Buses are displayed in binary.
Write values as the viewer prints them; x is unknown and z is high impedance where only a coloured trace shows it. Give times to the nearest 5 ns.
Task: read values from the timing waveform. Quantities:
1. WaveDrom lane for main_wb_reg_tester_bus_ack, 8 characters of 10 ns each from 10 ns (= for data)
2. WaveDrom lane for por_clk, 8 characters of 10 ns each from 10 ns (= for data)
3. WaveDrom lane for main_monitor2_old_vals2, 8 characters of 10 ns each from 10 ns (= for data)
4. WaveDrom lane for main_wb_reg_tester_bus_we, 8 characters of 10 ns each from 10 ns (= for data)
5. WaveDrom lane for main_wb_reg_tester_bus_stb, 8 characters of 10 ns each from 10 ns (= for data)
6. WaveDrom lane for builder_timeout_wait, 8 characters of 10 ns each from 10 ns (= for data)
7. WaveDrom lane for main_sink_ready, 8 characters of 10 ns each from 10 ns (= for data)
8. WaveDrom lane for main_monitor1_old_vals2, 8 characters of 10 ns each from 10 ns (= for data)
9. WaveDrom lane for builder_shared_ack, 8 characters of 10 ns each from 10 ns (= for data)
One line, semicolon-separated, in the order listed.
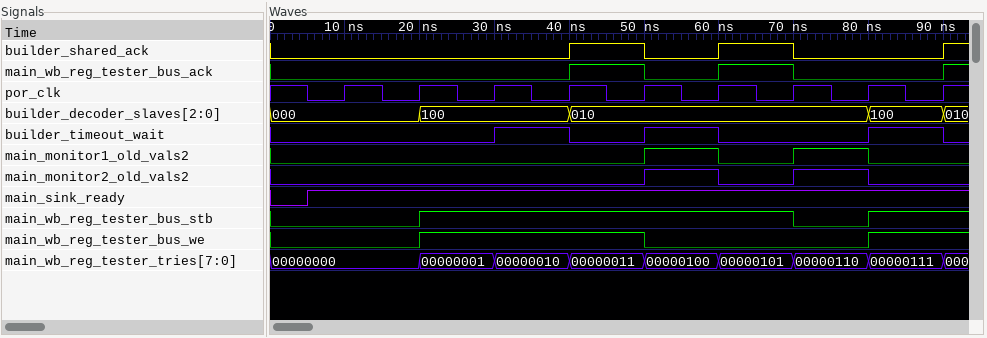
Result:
{name: 'main_wb_reg_tester_bus_ack', wave: '0..1010.'}; {name: 'por_clk', wave: 'p.......'}; {name: 'main_monitor2_old_vals2', wave: '0...1010'}; {name: 'main_wb_reg_tester_bus_we', wave: '01..0..1'}; {name: 'main_wb_reg_tester_bus_stb', wave: '01....01'}; {name: 'builder_timeout_wait', wave: '0.1010.1'}; {name: 'main_sink_ready', wave: '1.......'}; {name: 'main_monitor1_old_vals2', wave: '0...1010'}; {name: 'builder_shared_ack', wave: '0..1010.'}
